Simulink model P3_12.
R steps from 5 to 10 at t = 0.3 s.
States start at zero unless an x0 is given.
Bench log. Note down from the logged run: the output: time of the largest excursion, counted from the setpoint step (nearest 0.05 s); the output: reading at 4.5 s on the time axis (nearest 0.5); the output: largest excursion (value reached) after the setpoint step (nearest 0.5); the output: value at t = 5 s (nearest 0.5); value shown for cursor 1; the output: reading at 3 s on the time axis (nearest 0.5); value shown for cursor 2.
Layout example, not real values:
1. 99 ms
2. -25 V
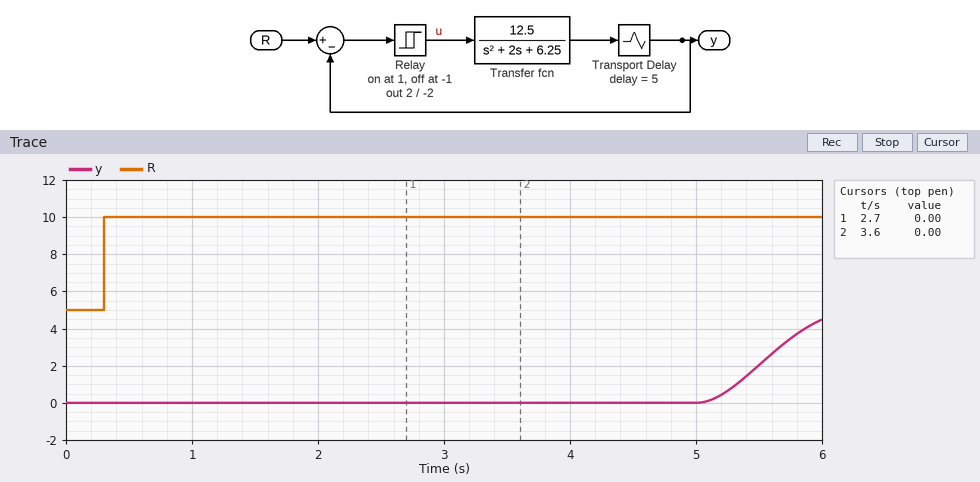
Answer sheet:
1. 5.70 s
2. 0.0
3. 4.5
4. 0.0
5. 0.00
6. 0.0
7. 0.00
